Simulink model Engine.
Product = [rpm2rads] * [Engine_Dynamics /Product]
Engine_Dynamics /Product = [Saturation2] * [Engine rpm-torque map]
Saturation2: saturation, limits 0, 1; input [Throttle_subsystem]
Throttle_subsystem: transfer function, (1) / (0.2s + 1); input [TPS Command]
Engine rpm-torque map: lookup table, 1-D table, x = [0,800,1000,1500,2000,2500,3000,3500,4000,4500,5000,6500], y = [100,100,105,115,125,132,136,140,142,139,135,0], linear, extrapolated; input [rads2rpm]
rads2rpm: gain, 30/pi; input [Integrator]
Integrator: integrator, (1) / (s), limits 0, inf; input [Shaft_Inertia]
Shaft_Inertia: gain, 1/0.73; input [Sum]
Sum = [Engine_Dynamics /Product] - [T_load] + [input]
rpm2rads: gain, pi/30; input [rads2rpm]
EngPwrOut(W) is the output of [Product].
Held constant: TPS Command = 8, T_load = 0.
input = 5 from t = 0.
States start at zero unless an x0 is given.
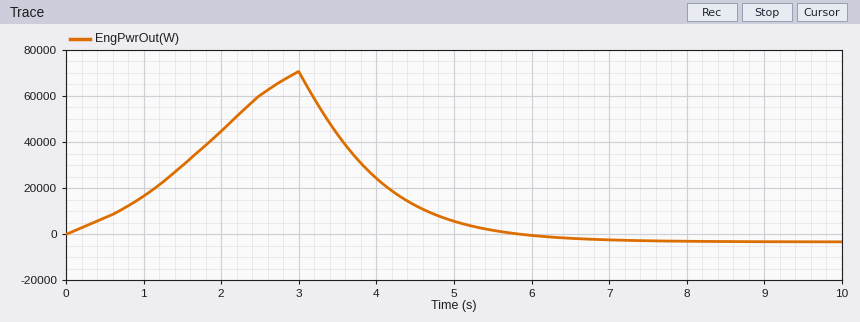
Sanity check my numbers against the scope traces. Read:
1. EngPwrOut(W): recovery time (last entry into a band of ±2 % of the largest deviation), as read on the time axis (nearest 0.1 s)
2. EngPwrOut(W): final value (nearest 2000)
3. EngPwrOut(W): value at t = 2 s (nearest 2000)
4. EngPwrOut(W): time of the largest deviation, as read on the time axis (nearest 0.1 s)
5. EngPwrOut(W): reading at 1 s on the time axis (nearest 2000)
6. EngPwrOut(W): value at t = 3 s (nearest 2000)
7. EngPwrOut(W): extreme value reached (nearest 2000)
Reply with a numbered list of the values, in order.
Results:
1. 6.6 s
2. -4000
3. 44000
4. 3.0 s
5. 16000
6. 70000
7. 70000
